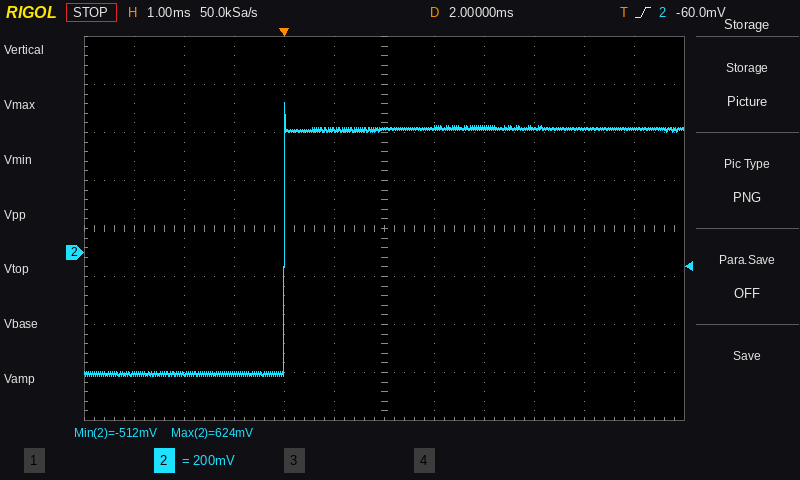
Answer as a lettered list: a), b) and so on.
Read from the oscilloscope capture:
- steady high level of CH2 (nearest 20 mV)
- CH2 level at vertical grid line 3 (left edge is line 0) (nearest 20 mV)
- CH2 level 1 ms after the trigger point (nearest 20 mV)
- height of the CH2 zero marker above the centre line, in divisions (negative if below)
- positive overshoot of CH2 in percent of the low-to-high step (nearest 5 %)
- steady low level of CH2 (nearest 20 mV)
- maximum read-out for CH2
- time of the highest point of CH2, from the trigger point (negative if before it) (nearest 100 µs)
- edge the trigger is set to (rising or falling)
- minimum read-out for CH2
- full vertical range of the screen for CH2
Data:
a) 520 mV
b) -500 mV
c) 520 mV
d) -0.5 div
e) 10 %
f) -500 mV
g) 624 mV
h) 0.0 ms
i) rising
j) -512 mV
k) 1.6 V
